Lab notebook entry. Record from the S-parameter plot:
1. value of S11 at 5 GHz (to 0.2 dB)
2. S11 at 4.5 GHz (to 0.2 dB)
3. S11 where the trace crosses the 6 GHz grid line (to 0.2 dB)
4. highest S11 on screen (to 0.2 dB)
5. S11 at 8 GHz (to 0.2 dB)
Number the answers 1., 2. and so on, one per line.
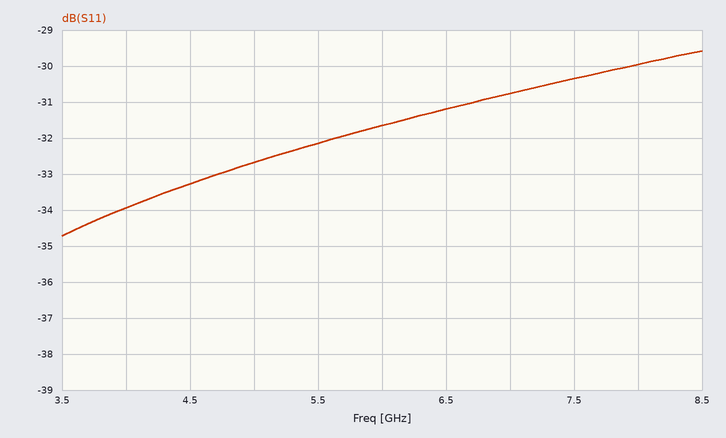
1. -32.6 dB
2. -33.2 dB
3. -31.6 dB
4. -29.6 dB
5. -30.0 dB
